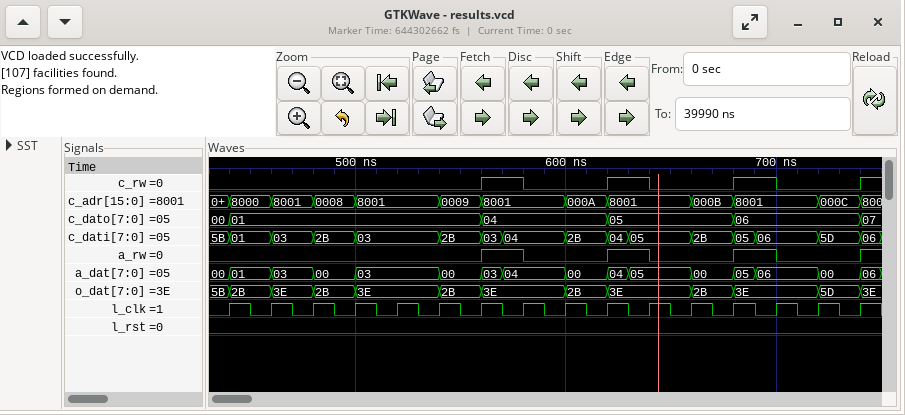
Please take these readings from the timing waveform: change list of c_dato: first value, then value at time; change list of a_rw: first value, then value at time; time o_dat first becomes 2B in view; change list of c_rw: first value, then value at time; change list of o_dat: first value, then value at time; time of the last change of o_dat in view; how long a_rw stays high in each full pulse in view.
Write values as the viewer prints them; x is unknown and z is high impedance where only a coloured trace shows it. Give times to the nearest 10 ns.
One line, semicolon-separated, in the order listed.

00, 01 at 440 ns, 04 at 560 ns, 05 at 620 ns, 06 at 680 ns, 07 at 740 ns; 0, 1 at 560 ns, 0 at 580 ns, 1 at 620 ns, 0 at 640 ns, 1 at 680 ns, 0 at 700 ns, 1 at 740 ns; 440 ns; 0, 1 at 560 ns, 0 at 580 ns, 1 at 620 ns, 0 at 640 ns, 1 at 680 ns, 0 at 700 ns, 1 at 740 ns; 5B, 2B at 440 ns, 3E at 460 ns, 2B at 480 ns, 3E at 500 ns, 2B at 540 ns, 3E at 560 ns, 2B at 600 ns, 3E at 620 ns, 2B at 660 ns, 3E at 680 ns, 5D at 720 ns, 3E at 740 ns; 740 ns; 20 ns, 20 ns, 20 ns
